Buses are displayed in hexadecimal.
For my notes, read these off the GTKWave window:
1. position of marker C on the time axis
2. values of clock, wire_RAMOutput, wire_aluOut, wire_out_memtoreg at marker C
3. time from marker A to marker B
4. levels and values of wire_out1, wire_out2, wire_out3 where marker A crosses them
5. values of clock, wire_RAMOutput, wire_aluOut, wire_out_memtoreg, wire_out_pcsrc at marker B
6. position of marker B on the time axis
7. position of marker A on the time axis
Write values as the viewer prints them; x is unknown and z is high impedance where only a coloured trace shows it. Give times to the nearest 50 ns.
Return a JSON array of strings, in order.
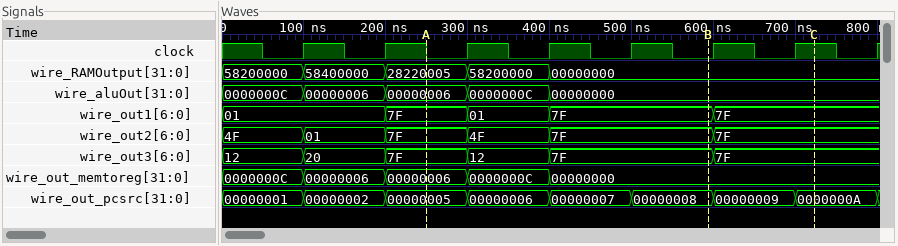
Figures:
["700 ns", "clock=1, wire_RAMOutput=00000000, wire_aluOut=00000000, wire_out_memtoreg=00000000", "350 ns", "wire_out1=7F, wire_out2=7F, wire_out3=7F", "clock=0, wire_RAMOutput=00000000, wire_aluOut=00000000, wire_out_memtoreg=00000000, wire_out_pcsrc=00000008", "600 ns", "250 ns"]
